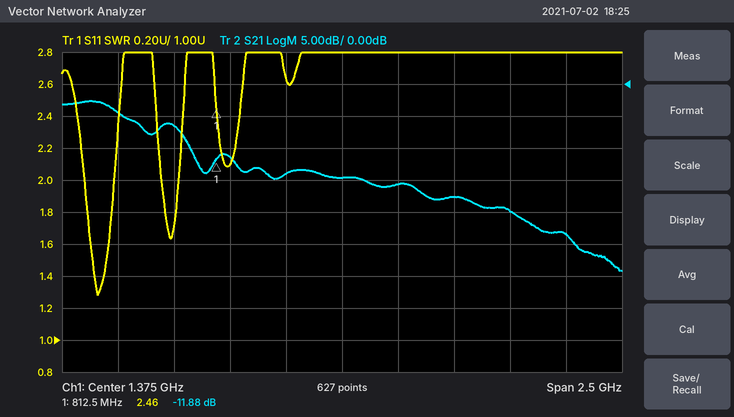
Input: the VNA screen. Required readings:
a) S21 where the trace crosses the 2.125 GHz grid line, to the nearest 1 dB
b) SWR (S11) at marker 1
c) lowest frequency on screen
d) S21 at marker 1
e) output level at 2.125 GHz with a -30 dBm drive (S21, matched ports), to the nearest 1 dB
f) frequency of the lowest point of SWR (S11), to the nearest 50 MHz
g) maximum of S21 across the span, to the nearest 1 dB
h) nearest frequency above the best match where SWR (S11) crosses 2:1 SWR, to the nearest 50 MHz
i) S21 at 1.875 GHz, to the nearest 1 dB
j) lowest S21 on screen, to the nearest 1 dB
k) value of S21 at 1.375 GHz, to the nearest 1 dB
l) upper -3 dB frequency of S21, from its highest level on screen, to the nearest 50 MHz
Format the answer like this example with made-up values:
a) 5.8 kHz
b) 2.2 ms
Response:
a) -20 dB
b) 2.46
c) 125 MHz
d) -11.88 dB
e) -50 dBm
f) 300 MHz
g) -3 dB
h) 350 MHz
i) -18 dB
j) -29 dB
k) -15 dB
l) 450 MHz
